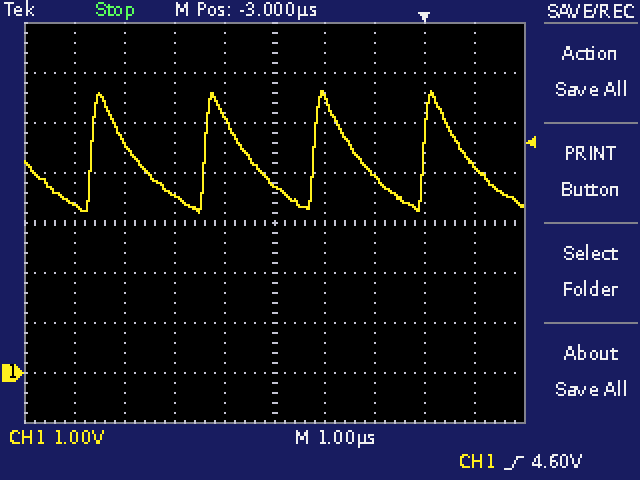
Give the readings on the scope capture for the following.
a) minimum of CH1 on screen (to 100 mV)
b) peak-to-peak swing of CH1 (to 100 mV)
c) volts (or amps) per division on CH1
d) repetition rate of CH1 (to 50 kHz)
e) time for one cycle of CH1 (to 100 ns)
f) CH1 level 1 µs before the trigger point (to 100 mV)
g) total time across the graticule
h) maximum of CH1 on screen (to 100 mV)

3.2 V
2.4 V
1 V
450 kHz
2.2 µs
4.0 V
10 µs
5.6 V
